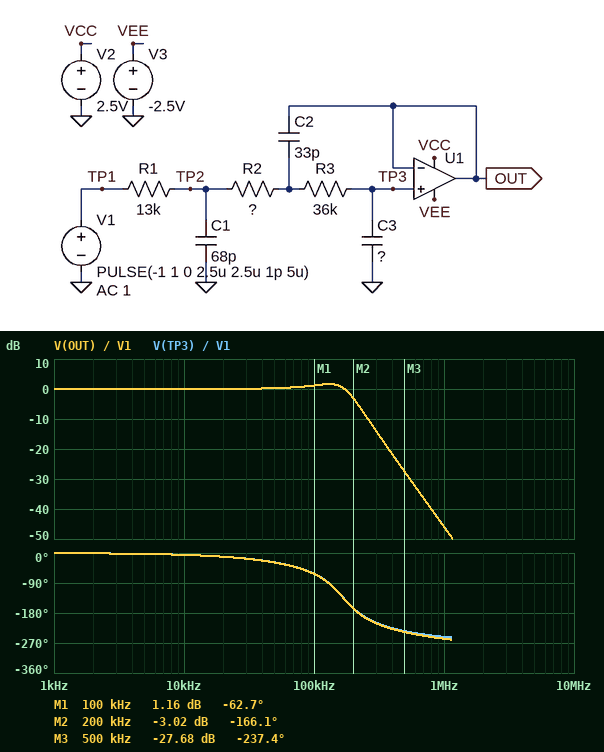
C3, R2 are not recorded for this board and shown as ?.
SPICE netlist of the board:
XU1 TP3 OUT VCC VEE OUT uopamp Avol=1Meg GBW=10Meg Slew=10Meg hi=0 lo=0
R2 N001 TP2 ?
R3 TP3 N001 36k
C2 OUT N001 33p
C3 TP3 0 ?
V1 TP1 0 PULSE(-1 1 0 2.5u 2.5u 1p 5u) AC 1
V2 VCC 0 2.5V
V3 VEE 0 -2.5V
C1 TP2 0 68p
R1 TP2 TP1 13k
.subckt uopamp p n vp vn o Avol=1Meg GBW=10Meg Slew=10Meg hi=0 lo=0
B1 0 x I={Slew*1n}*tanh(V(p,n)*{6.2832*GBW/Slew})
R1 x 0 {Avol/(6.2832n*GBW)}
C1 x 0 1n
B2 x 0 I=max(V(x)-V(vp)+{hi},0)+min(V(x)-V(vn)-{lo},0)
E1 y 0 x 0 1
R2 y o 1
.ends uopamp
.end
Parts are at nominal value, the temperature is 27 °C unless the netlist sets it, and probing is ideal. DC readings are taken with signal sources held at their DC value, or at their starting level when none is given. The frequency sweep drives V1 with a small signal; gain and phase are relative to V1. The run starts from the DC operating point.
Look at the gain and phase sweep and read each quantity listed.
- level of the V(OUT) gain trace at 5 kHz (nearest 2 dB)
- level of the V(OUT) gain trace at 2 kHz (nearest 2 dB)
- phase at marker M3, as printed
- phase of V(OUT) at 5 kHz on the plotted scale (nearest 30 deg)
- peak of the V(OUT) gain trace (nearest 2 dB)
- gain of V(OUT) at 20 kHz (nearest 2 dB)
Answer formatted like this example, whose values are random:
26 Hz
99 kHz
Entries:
0 dB
0 dB
-237.4 deg
0 deg
2 dB
0 dB
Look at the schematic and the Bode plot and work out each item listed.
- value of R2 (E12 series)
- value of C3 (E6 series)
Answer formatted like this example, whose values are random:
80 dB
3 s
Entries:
390 kΩ
1.5 pF
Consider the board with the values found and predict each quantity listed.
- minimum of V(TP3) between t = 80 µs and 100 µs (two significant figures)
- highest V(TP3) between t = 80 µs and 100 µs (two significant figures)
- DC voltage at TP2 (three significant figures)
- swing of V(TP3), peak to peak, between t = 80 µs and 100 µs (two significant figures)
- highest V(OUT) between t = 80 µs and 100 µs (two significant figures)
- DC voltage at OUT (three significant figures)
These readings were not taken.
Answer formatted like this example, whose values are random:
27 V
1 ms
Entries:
-570 mV
570 mV
-1.00 V
1.1 V
570 mV
-1.00 V
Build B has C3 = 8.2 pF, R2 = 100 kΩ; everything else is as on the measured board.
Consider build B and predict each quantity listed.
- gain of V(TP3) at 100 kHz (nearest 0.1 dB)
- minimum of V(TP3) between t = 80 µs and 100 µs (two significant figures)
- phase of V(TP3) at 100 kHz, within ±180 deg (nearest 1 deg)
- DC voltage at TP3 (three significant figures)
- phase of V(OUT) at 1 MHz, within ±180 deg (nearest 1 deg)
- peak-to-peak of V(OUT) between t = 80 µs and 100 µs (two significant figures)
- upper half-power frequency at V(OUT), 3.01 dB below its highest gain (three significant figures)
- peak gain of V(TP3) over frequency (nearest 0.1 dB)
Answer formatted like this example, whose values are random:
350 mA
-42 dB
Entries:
-0.9 dB
-320 mV
-82 deg
-1.00 V
106 deg
640 mV
141 kHz
0 dB
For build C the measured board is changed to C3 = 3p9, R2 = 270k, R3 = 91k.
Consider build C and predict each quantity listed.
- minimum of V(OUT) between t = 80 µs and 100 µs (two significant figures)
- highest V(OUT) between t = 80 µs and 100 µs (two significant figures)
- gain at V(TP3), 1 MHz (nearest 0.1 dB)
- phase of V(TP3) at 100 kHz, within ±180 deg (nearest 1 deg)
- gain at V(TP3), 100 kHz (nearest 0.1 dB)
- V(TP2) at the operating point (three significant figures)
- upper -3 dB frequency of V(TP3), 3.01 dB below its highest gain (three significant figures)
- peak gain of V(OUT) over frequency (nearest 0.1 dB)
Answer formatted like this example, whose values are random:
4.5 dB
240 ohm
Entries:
-120 mV
120 mV
-57.3 dB
-139 deg
-1.1 dB
-1.00 V
98.8 kHz
2.1 dB
